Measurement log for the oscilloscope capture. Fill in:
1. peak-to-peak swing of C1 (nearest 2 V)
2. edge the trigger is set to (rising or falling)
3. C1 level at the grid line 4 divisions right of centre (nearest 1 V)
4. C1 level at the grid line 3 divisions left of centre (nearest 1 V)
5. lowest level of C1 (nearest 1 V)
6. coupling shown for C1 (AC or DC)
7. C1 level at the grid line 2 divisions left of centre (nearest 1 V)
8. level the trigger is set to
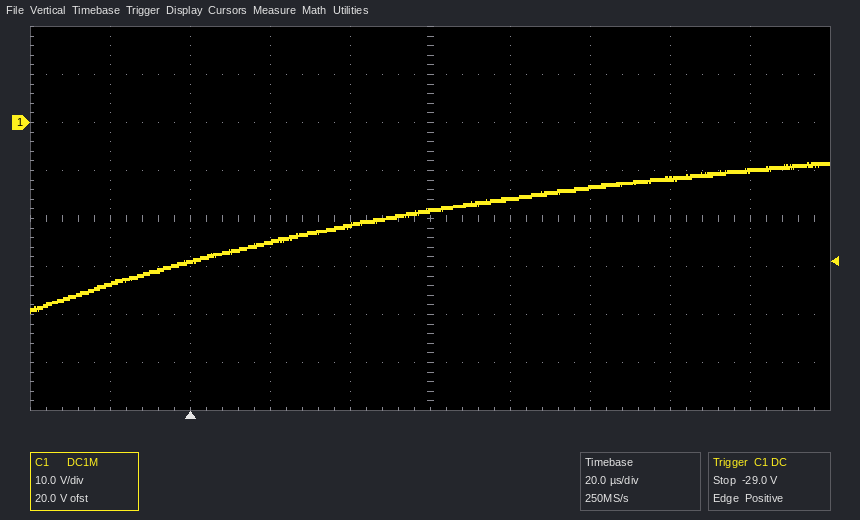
32 V
rising
-10 V
-29 V
-40 V
DC
-25 V
-29.0 V
